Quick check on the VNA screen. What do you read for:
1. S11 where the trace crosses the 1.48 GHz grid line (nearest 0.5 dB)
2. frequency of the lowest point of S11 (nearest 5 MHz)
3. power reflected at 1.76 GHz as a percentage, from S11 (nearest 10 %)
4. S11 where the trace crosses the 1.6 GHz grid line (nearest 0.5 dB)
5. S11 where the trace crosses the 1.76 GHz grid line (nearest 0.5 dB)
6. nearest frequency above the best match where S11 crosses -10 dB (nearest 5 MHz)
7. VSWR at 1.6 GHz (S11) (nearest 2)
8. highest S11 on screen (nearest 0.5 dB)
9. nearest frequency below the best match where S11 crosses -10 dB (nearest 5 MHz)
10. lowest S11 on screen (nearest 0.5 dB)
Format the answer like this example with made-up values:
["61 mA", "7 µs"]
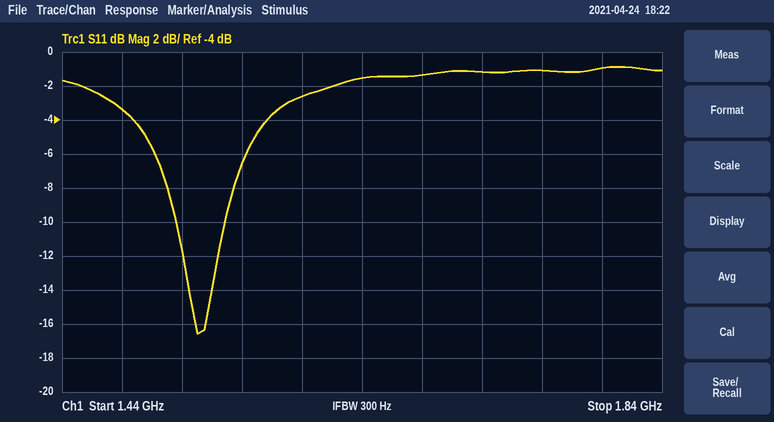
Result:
["-3.5 dB", "1.530 GHz", "80 %", "-2.5 dB", "-1.0 dB", "1.550 GHz", "6", "-1.0 dB", "1.515 GHz", "-16.5 dB"]
